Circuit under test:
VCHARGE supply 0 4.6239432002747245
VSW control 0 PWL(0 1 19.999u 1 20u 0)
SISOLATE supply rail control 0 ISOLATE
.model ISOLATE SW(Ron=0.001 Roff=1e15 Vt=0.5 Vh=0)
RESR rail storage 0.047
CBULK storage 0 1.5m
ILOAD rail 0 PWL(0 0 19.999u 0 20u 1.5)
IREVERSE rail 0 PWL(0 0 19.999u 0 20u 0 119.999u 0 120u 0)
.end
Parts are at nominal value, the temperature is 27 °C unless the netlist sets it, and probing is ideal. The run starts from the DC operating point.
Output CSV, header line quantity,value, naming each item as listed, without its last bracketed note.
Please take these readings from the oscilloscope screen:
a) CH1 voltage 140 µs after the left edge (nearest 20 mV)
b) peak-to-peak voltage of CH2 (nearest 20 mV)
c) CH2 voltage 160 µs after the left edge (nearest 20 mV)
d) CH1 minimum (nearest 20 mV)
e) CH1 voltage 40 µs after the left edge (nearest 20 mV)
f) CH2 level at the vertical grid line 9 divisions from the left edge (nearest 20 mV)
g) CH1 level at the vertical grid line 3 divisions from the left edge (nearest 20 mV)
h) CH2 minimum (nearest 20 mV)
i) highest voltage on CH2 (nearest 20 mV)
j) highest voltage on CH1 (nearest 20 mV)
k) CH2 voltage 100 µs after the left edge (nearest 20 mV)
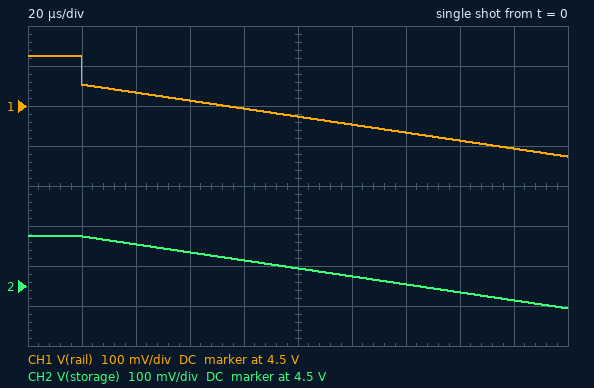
quantity,value
CH1 voltage 140 µs after the left edge,4.44 V
peak-to-peak voltage of CH2,180 mV
CH2 voltage 160 µs after the left edge,4.48 V
CH1 minimum,4.38 V
CH1 voltage 40 µs after the left edge,4.54 V
CH2 level at the vertical grid line 9 divisions from the left edge,4.46 V
CH1 level at the vertical grid line 3 divisions from the left edge,4.52 V
CH2 minimum,4.44 V
highest voltage on CH2,4.62 V
highest voltage on CH1,4.62 V
CH2 voltage 100 µs after the left edge,4.54 V
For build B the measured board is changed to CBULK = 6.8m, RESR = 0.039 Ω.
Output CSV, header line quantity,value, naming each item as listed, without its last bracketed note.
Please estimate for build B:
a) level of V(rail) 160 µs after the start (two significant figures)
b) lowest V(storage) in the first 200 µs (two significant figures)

quantity,value
level of V(rail) 160 µs after the start,4.5 V
lowest V(storage) in the first 200 µs,4.6 V
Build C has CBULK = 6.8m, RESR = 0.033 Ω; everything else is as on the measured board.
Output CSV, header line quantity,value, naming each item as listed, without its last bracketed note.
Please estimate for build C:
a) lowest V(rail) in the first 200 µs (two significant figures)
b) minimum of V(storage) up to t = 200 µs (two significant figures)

quantity,value
lowest V(rail) in the first 200 µs,4.5 V
minimum of V(storage) up to t = 200 µs,4.6 V
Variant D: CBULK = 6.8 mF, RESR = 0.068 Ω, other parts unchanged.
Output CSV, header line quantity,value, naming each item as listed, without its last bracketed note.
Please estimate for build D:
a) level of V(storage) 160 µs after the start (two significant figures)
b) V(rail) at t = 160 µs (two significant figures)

quantity,value
level of V(storage) 160 µs after the start,4.6 V
V(rail) at t = 160 µs,4.5 V
